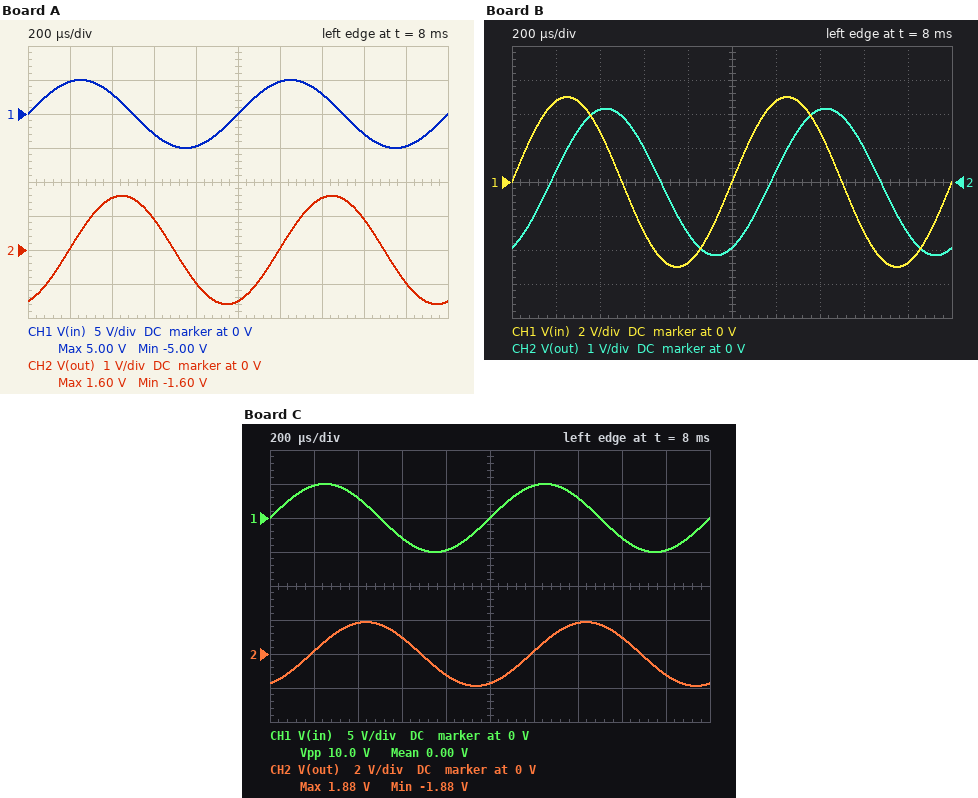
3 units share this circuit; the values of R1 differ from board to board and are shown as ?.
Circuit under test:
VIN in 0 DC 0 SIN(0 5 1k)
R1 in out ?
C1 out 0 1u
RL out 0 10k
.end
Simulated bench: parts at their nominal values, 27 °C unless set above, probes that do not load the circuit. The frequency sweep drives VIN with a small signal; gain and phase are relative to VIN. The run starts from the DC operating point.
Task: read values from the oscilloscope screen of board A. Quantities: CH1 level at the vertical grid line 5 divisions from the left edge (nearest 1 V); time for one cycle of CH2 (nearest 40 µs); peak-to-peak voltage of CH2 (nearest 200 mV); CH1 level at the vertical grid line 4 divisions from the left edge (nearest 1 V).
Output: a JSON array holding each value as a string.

["0 V", "1.00 ms", "3.2 V", "-5 V"]
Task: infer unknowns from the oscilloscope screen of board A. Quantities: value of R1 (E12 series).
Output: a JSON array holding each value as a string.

["470 Ω"]
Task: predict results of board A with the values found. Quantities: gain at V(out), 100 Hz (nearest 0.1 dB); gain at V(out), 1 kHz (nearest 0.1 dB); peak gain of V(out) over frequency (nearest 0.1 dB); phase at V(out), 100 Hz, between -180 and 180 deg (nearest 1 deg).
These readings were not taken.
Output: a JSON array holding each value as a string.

["-0.7 dB", "-9.9 dB", "-0.4 dB", "-16 deg"]
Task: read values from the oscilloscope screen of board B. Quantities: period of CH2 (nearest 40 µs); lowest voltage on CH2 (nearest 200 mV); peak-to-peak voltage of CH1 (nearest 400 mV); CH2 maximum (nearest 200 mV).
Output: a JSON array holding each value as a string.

["1.00 ms", "-2.2 V", "10.0 V", "2.2 V"]
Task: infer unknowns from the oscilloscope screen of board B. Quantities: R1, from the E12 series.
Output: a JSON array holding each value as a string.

["330 Ω"]
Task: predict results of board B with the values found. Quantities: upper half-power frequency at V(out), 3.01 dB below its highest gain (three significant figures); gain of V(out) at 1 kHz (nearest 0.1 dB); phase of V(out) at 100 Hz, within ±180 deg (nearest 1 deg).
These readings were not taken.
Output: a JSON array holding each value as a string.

["498 Hz", "-7.3 dB", "-11 deg"]
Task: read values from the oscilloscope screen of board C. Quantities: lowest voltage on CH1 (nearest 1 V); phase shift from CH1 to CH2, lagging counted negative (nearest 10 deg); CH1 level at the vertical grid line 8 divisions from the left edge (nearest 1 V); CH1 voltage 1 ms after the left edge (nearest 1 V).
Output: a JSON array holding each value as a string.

["-5 V", "-70 deg", "-3 V", "0 V"]
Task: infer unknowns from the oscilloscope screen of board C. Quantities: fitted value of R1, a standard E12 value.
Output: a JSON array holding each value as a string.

["390 Ω"]
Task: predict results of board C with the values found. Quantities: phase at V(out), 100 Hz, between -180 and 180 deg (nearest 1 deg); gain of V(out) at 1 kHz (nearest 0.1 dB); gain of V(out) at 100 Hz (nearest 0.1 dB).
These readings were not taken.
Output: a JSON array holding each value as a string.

["-13 deg", "-8.5 dB", "-0.6 dB"]
